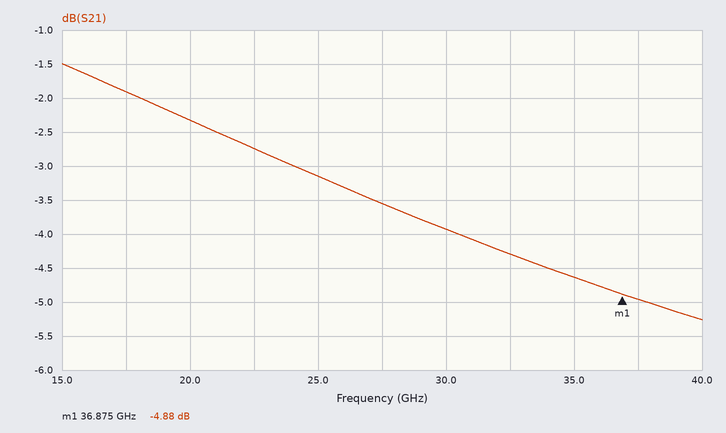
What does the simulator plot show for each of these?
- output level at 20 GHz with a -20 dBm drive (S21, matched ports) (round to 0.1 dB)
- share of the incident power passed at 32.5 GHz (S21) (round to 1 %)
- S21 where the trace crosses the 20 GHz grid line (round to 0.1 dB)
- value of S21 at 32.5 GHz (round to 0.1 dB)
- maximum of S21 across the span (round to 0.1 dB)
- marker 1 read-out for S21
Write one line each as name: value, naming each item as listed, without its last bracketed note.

output level at 20 GHz with a -20 dBm drive (S21, matched ports): -22.3 dBm
share of the incident power passed at 32.5 GHz (S21): 37 %
S21 where the trace crosses the 20 GHz grid line: -2.3 dB
value of S21 at 32.5 GHz: -4.3 dB
maximum of S21 across the span: -1.5 dB
marker 1 read-out for S21: -4.88 dB
